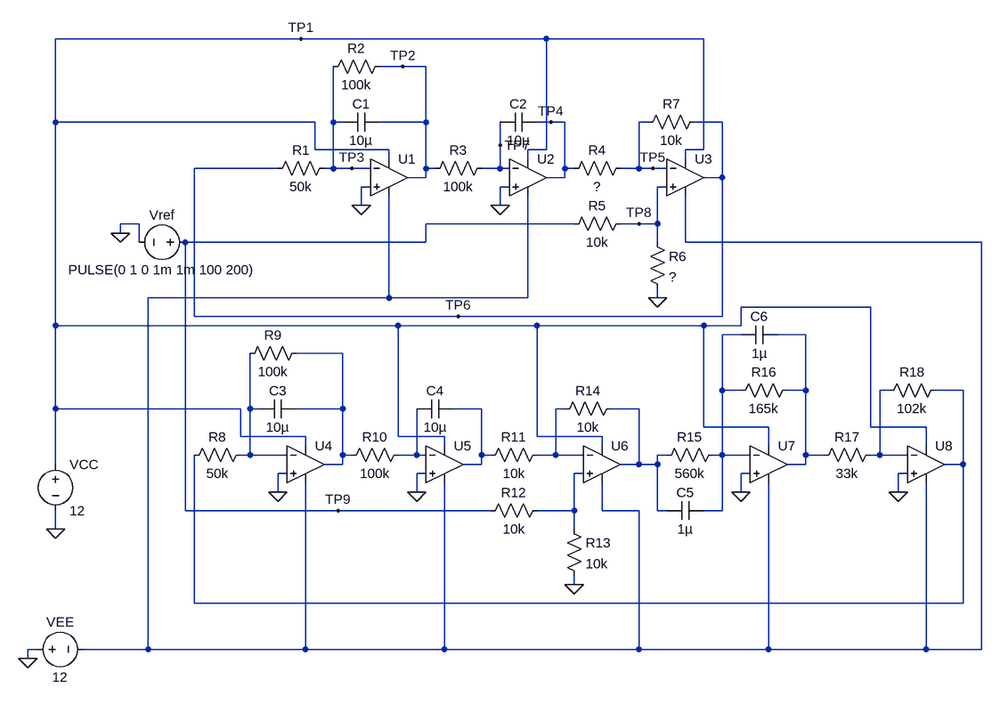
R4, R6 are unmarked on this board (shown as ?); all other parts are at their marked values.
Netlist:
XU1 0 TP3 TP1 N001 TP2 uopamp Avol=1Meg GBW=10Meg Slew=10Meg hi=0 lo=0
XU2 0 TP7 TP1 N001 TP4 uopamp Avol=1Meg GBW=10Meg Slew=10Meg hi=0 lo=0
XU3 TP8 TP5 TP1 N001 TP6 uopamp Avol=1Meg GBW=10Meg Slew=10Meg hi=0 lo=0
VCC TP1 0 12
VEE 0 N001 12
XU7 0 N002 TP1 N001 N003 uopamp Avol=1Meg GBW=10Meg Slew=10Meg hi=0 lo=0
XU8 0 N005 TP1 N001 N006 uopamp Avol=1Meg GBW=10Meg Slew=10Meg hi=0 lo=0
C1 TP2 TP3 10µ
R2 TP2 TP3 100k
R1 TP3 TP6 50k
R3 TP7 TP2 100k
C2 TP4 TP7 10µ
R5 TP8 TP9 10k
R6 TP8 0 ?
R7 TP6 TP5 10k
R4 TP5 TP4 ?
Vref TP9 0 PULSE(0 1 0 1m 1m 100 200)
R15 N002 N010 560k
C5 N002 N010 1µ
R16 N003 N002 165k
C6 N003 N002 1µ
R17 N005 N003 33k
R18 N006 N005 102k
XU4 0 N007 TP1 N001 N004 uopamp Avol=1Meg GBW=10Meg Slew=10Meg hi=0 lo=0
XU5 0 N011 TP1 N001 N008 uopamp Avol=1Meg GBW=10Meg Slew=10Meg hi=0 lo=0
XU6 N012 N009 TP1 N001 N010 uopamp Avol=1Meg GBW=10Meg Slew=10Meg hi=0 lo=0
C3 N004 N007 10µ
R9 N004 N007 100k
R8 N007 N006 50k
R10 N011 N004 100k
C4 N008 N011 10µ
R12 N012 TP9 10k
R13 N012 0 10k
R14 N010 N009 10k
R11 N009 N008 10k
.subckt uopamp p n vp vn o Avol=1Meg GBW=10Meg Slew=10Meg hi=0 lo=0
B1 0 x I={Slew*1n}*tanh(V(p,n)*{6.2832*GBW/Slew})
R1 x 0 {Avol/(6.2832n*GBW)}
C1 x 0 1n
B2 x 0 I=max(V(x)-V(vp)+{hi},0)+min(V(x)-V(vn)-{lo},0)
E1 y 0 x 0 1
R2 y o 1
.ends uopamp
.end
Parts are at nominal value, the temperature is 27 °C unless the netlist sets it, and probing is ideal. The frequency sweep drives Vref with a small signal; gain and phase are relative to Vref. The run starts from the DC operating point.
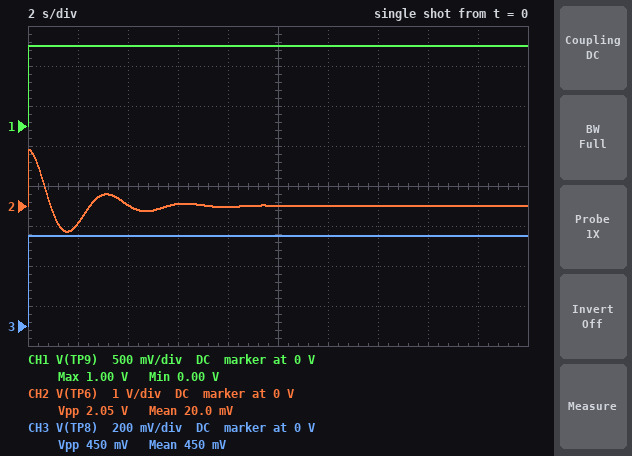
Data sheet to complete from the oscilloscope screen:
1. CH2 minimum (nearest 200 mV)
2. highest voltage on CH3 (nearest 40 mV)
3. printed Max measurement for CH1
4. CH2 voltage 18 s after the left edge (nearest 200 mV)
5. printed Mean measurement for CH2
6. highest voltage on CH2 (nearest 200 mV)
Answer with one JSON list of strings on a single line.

["-600 mV", "440 mV", "1.00 V", "0 V", "20.0 mV", "1.4 V"]
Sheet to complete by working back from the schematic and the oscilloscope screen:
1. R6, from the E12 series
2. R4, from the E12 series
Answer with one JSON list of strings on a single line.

["8.2 kΩ", "4.7 kΩ"]
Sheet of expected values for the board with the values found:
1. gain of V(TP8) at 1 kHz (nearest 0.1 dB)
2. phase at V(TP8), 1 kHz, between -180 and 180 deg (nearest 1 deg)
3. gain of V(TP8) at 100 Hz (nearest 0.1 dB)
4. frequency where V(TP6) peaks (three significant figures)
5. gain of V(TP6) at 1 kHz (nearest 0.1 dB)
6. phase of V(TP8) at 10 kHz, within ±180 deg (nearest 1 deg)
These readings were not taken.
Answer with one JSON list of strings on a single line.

["-6.9 dB", "0 deg", "-6.9 dB", "345 mHz", "3.0 dB", "0 deg"]
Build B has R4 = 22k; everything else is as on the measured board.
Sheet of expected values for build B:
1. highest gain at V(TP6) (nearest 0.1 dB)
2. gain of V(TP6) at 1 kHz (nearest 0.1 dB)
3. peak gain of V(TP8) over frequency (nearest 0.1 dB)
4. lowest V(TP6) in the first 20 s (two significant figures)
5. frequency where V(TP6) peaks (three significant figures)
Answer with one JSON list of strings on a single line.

["-0.5 dB", "-3.7 dB", "-6.9 dB", "-95 mV", "179 mHz"]
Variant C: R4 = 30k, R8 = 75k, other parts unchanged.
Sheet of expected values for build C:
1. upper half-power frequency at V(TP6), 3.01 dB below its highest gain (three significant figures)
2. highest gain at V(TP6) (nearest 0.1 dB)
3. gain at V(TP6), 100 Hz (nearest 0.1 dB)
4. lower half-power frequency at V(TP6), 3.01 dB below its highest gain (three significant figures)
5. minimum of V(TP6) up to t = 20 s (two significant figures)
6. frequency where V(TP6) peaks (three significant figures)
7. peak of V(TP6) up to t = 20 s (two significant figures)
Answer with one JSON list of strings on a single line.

["2.50 MHz", "-1.9 dB", "-4.4 dB", "87.3 mHz", "-53 mV", "159 mHz", "600 mV"]
